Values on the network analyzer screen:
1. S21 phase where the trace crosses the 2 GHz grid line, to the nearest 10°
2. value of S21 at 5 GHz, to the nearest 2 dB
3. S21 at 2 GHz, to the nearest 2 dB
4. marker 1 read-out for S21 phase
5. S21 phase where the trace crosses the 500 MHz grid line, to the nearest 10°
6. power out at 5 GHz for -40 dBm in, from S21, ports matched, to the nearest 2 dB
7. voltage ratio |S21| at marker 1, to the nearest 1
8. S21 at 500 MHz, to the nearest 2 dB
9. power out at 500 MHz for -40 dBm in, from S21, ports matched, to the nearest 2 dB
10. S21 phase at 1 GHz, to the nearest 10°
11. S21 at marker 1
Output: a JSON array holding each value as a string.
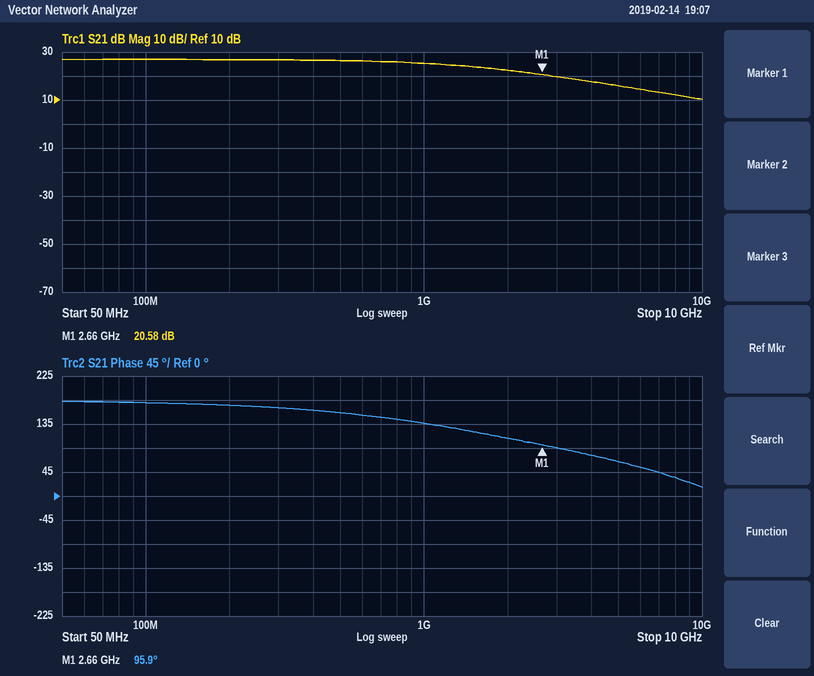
["110°", "16 dB", "22 dB", "95.9°", "160°", "-24 dBm", "11", "26 dB", "-14 dBm", "140°", "20.58 dB"]
